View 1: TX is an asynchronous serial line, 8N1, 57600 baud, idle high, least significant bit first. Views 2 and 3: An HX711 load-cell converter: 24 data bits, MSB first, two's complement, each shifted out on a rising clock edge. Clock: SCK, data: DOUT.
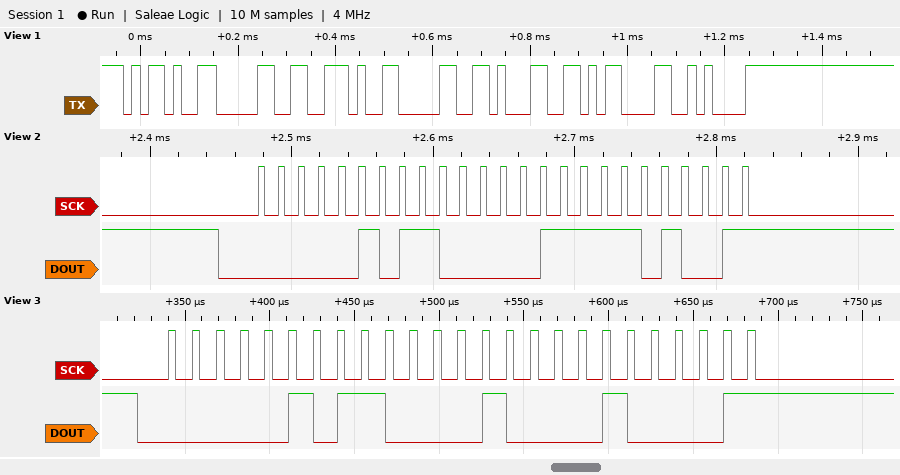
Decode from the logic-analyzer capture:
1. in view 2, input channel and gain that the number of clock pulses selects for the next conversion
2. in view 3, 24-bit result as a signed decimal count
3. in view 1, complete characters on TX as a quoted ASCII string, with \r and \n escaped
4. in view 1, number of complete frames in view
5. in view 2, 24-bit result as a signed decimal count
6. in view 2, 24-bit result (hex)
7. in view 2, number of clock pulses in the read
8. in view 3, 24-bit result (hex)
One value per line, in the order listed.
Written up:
channel A, gain 128
361505
"-0.01\r\n"
7
361449
0x0583E9
25
0x058421
